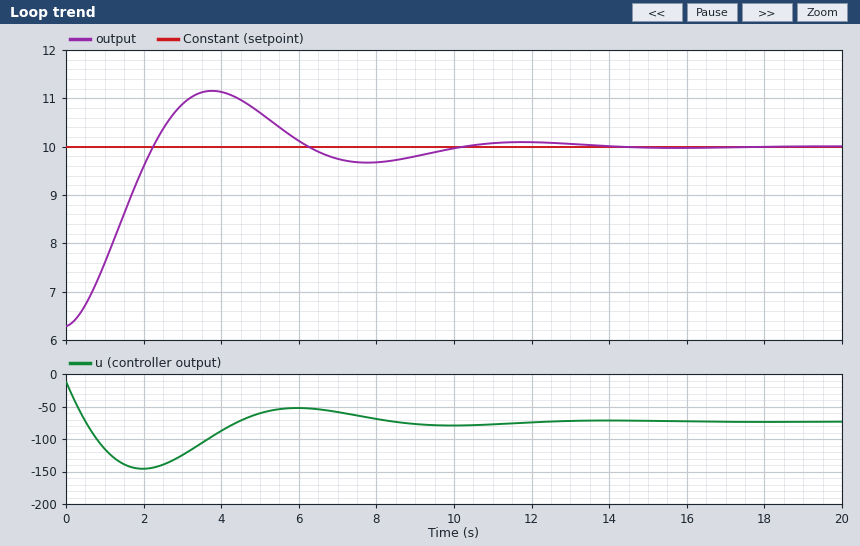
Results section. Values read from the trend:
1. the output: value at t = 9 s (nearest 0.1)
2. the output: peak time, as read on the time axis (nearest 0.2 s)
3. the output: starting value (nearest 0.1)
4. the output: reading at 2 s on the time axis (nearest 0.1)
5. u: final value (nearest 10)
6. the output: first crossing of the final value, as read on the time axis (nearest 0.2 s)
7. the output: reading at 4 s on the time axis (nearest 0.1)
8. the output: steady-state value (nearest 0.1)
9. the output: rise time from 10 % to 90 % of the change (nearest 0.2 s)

9.8
3.8 s
6.3
9.6
-70
2.2 s
11.1
10.0
1.6 s
